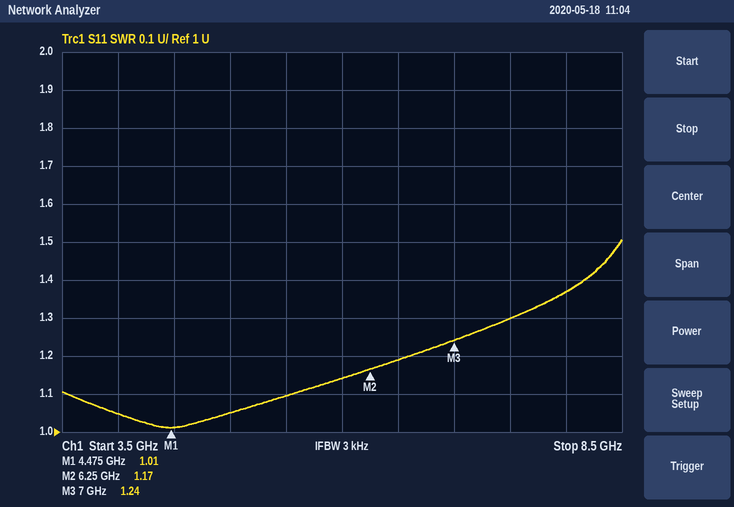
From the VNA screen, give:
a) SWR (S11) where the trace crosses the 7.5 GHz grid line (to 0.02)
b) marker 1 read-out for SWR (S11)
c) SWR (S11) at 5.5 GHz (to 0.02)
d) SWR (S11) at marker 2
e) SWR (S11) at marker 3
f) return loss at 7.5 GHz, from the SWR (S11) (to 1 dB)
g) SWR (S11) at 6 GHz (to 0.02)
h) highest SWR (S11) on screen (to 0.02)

1.30
1.01
1.10
1.17
1.24
18 dB
1.14
1.50
